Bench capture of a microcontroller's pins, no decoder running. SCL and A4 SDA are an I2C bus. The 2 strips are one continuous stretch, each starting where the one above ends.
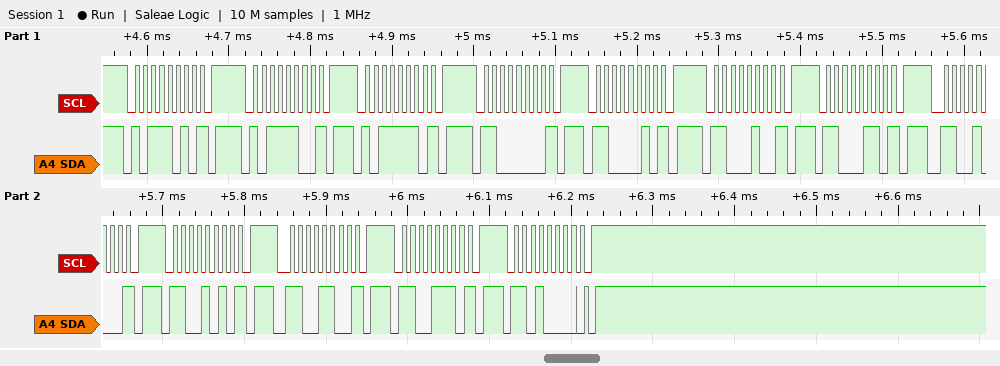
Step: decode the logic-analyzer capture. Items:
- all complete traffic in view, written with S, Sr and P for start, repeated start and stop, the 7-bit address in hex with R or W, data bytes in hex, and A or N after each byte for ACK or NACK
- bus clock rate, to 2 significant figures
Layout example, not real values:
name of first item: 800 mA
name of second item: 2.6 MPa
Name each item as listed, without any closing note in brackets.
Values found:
all complete traffic in view, written with S, Sr and P for start, repeated start and stop, the 7-bit address in hex with R or W, data bytes in hex, and A or N after each byte for ACK or NACK: S 5DW N P S 5EW N P S 5FW N P S 60W N P S 61W N P S 62W N P S 63W N P S 64W N P S 65W N P S 66W N P S 67W N P S 68W A P
bus clock rate, to 2 significant figures: 100 kHz
